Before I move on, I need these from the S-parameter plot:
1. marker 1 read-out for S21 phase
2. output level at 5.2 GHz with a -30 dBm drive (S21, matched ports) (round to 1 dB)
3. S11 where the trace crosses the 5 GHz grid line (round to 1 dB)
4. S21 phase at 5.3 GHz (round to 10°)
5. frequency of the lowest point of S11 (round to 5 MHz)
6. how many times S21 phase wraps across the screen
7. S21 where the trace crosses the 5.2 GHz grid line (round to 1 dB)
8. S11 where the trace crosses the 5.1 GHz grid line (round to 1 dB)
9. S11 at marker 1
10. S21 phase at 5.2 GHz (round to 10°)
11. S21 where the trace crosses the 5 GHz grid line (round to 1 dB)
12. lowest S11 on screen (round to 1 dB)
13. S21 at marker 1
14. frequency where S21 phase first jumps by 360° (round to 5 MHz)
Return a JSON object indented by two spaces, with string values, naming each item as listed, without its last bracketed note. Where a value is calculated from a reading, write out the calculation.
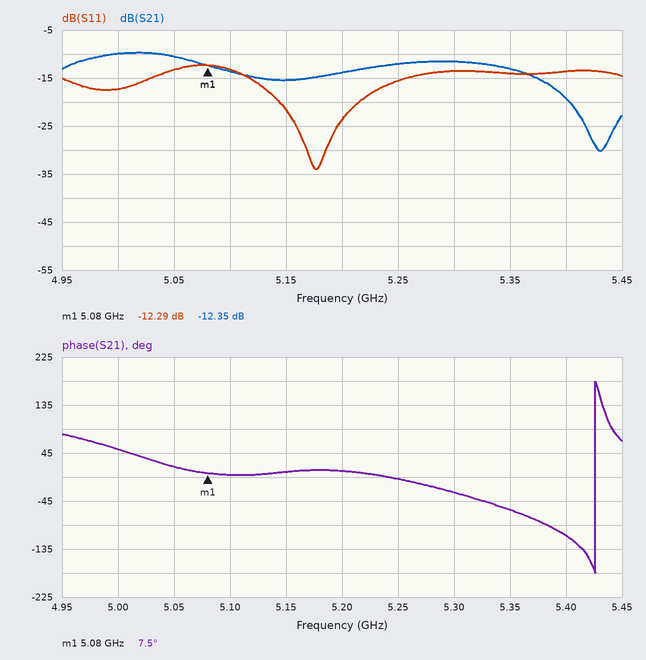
{
  "marker 1 read-out for S21 phase": "7.5°",
  "output level at 5.2 GHz with a -30 dBm drive (S21, matched ports)": "-30 dBm + (-14 dB) = -44 dBm",
  "S11 where the trace crosses the 5 GHz grid line": "-17 dB",
  "S21 phase at 5.3 GHz": "-30°",
  "frequency of the lowest point of S11": "5.175 GHz",
  "how many times S21 phase wraps across the screen": "1",
  "S21 where the trace crosses the 5.2 GHz grid line": "-14 dB",
  "S11 where the trace crosses the 5.1 GHz grid line": "-13 dB",
  "S11 at marker 1": "-12.29 dB",
  "S21 phase at 5.2 GHz": "10°",
  "S21 where the trace crosses the 5 GHz grid line": "-10 dB",
  "lowest S11 on screen": "-34 dB",
  "S21 at marker 1": "-12.35 dB",
  "frequency where S21 phase first jumps by 360°": "5.425 GHz"
}
